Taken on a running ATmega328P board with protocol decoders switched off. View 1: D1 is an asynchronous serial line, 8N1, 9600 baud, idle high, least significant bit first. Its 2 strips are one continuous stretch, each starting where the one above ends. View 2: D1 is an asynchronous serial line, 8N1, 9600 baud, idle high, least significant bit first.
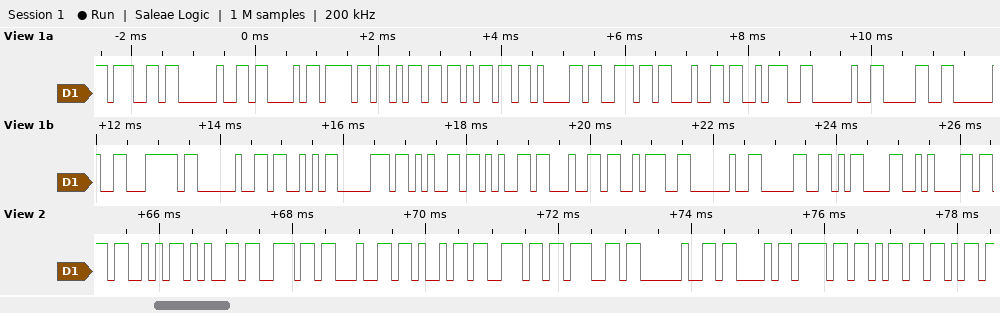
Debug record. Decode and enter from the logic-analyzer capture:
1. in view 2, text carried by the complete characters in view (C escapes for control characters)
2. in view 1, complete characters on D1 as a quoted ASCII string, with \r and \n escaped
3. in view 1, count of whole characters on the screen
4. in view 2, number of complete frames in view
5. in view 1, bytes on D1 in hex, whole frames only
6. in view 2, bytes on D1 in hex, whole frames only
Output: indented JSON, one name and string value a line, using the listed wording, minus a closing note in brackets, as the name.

{
  "in view 2, text carried by the complete characters in view": "\"Sending Com\"",
  "in view 1, complete characters on D1 as a quoted ASCII string, with \\r and \\n escaped": "\"g Command: 0 | Speed: 0\\r\\n\"",
  "in view 1, count of whole characters on the screen": "25",
  "in view 2, number of complete frames in view": "11",
  "in view 1, bytes on D1 in hex, whole frames only": "67 20 43 6F 6D 6D 61 6E 64 3A 20 30 20 7C 20 53 70 65 65 64 3A 20 30 0D 0A",
  "in view 2, bytes on D1 in hex, whole frames only": "53 65 6E 64 69 6E 67 20 43 6F 6D"
}
